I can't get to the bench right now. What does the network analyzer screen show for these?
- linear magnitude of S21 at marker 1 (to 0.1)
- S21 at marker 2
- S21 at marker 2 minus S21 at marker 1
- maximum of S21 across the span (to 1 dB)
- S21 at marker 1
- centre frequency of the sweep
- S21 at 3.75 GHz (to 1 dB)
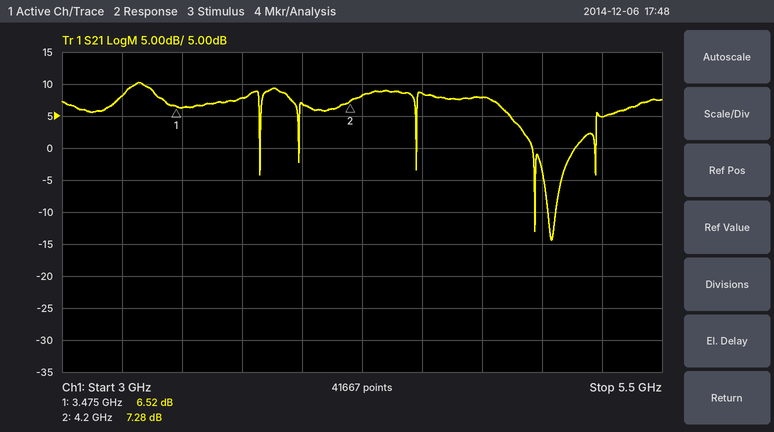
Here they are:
2.1
7.28 dB
0.76 dB
10 dB
6.52 dB
4.25 GHz
8 dB
